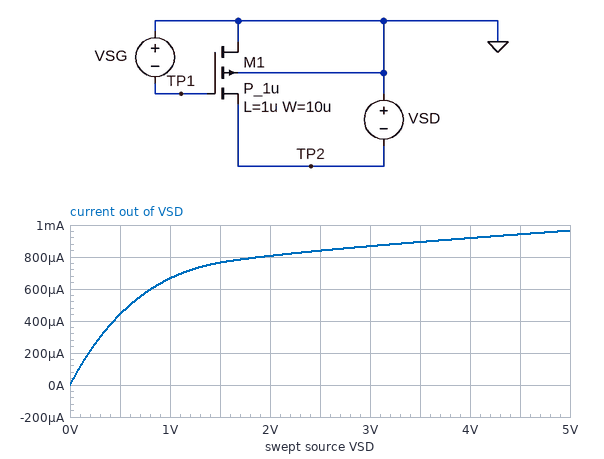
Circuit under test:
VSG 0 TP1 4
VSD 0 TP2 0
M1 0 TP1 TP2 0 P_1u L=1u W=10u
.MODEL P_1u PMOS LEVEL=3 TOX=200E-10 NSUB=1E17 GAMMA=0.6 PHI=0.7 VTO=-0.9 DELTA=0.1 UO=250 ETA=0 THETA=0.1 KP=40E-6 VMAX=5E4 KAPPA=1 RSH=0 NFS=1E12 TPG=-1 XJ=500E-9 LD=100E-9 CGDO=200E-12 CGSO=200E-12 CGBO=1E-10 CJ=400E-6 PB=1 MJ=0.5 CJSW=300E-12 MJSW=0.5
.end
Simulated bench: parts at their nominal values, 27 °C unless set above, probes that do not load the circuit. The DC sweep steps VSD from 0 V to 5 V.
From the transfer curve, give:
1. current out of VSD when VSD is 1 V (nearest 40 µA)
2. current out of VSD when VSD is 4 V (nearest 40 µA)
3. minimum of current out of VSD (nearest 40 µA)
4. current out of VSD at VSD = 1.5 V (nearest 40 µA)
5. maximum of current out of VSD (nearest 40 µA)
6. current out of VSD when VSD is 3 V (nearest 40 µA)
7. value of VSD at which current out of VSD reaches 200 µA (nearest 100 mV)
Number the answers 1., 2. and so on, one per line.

1. 680 µA
2. 920 µA
3. 0 A
4. 760 µA
5. 960 µA
6. 880 µA
7. 200 mV
